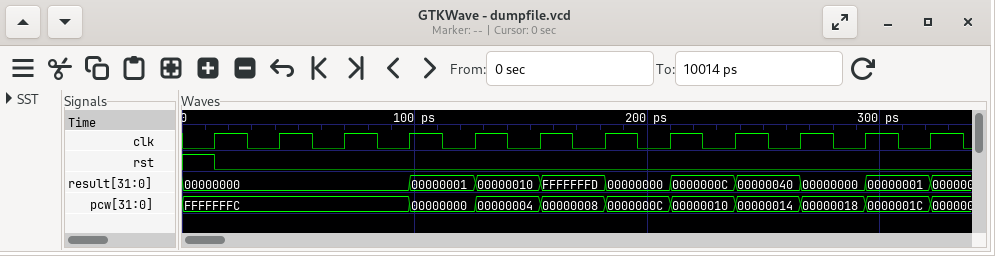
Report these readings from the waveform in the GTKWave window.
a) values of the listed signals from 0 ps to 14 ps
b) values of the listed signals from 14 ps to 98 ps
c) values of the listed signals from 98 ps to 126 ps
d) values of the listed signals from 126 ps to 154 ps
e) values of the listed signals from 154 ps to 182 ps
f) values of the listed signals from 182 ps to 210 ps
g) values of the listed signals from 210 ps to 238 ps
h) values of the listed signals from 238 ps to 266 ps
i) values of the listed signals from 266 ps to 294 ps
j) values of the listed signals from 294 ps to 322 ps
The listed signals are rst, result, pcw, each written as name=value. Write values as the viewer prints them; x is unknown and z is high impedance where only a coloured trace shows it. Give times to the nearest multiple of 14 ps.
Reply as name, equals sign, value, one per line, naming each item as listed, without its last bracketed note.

values of the listed signals from 0 ps to 14 ps = rst=1, result=00000000, pcw=FFFFFFFC
values of the listed signals from 14 ps to 98 ps = rst=0, result=00000000, pcw=FFFFFFFC
values of the listed signals from 98 ps to 126 ps = rst=0, result=00000001, pcw=00000000
values of the listed signals from 126 ps to 154 ps = rst=0, result=00000010, pcw=00000004
values of the listed signals from 154 ps to 182 ps = rst=0, result=FFFFFFFD, pcw=00000008
values of the listed signals from 182 ps to 210 ps = rst=0, result=00000000, pcw=0000000C
values of the listed signals from 210 ps to 238 ps = rst=0, result=0000000C, pcw=00000010
values of the listed signals from 238 ps to 266 ps = rst=0, result=00000040, pcw=00000014
values of the listed signals from 266 ps to 294 ps = rst=0, result=00000000, pcw=00000018
values of the listed signals from 294 ps to 322 ps = rst=0, result=00000001, pcw=0000001C
